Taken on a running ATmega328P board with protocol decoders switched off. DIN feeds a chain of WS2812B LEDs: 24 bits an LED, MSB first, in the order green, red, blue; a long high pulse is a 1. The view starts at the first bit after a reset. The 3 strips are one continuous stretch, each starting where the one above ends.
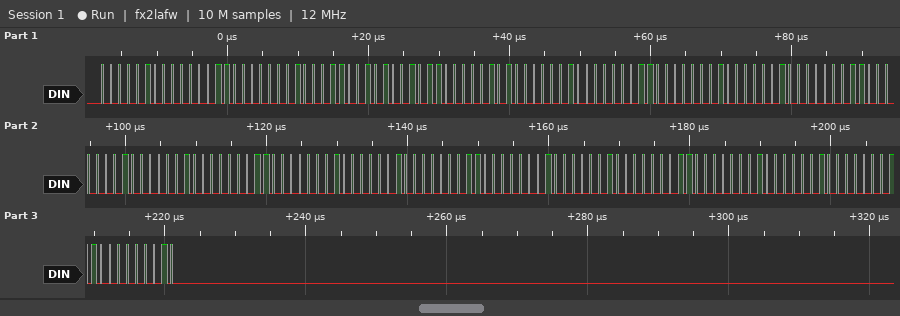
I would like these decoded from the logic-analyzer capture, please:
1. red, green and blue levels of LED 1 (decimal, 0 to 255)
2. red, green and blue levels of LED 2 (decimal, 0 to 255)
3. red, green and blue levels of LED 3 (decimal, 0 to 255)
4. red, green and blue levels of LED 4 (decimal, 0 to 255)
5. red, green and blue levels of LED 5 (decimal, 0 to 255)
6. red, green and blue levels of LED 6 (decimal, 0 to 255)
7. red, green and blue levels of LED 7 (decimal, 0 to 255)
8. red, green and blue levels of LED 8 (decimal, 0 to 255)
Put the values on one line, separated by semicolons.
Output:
6, 4, 2; 150, 50, 10; 6, 4, 2; 6, 4, 2; 6, 4, 2; 6, 4, 2; 6, 4, 2; 6, 4, 2
